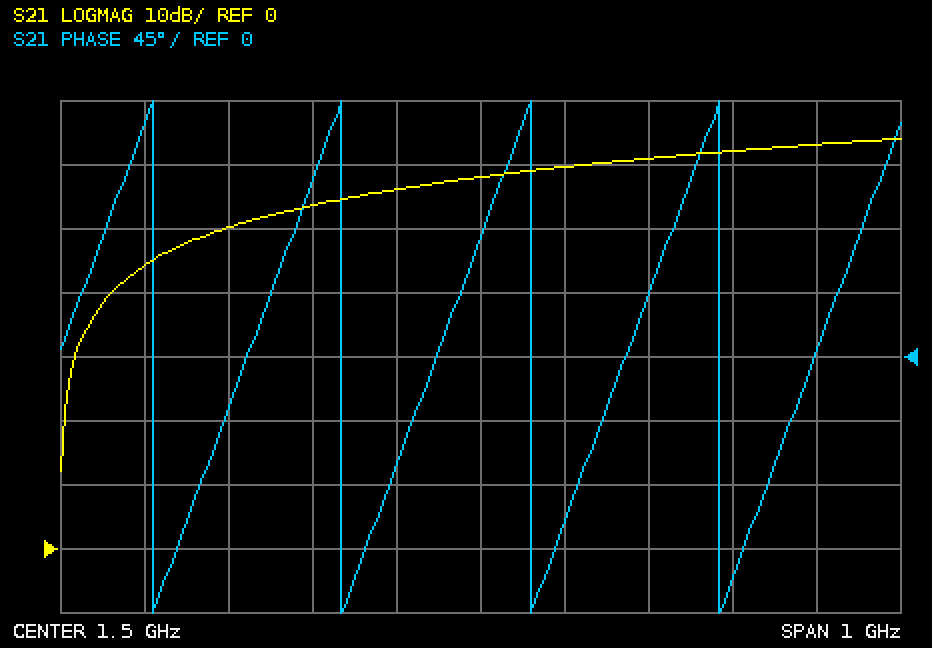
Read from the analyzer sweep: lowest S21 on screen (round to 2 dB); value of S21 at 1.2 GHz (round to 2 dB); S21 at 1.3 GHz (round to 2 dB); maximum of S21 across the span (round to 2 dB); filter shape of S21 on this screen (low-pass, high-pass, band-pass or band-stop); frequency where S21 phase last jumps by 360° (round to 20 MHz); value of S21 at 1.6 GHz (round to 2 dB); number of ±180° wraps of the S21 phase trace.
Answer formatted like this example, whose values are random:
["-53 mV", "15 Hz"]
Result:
["12 dB", "50 dB", "54 dB", "64 dB", "high-pass", "1.78 GHz", "60 dB", "4"]
